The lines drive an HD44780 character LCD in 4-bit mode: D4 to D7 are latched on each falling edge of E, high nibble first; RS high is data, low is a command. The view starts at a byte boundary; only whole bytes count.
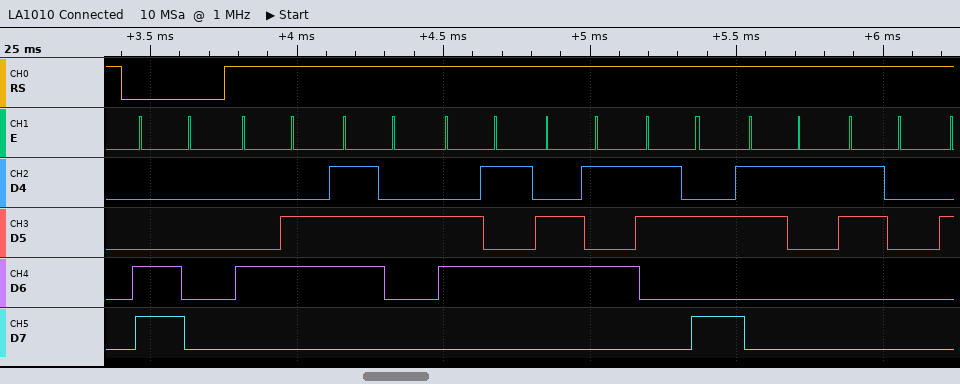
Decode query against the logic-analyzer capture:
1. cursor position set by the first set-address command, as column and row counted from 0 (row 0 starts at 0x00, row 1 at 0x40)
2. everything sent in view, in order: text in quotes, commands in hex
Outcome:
column 0, row 1
0xC0 "Free:10"
